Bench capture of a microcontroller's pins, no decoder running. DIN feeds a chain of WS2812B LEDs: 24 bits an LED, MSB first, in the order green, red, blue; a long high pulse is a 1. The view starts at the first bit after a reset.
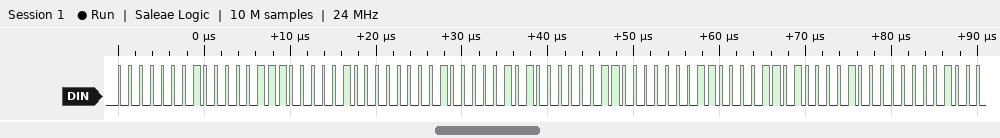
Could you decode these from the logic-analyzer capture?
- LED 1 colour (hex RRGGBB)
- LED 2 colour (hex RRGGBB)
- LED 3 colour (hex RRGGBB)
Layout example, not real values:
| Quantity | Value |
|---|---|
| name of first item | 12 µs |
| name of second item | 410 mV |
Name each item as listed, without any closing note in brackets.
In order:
| Quantity | Value |
|---|---|
| LED 1 colour | #070104 |
| LED 2 colour | #0A0206 |
| LED 3 colour | #0D0308 |
